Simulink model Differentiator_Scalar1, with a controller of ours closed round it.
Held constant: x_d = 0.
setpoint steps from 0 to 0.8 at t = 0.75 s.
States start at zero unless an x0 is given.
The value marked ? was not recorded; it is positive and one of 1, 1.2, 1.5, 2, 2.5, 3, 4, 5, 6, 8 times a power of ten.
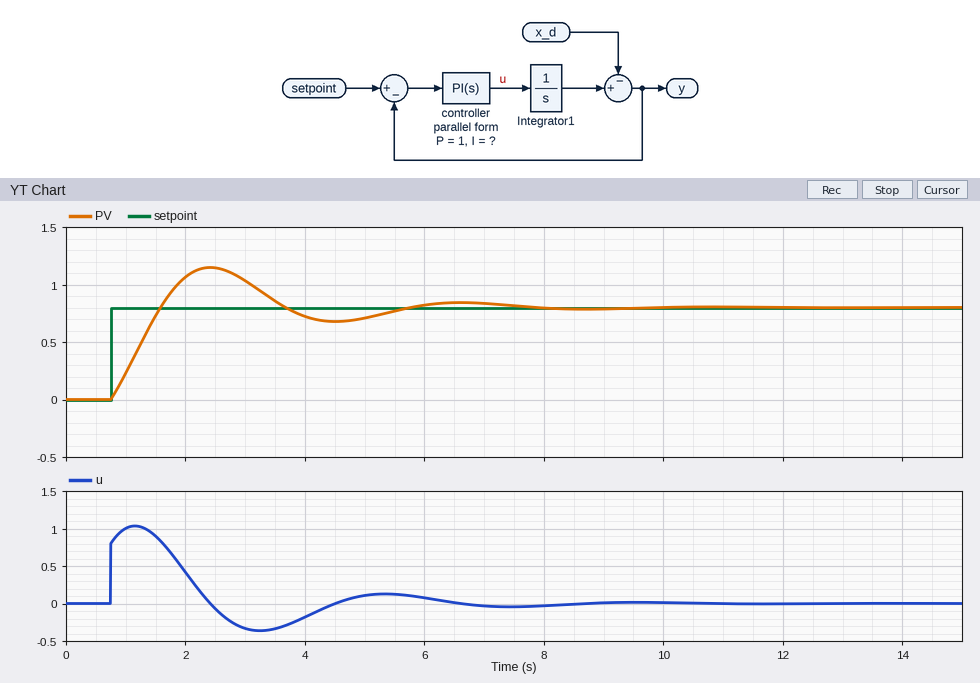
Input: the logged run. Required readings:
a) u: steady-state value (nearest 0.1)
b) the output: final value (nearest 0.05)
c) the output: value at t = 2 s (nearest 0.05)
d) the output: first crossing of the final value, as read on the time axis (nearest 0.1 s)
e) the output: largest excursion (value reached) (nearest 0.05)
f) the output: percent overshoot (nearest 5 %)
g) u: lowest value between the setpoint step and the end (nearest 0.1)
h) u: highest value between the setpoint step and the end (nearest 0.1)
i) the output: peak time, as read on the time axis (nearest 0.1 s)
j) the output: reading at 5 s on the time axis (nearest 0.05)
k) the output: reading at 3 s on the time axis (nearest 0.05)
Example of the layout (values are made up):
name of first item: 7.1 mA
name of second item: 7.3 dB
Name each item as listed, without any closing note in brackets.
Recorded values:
u: steady-state value: 0.0
the output: final value: 0.80
the output: value at t = 2 s: 1.05
the output: first crossing of the final value, as read on the time axis: 1.6 s
the output: largest excursion (value reached): 1.15
the output: percent overshoot: 45 %
u: lowest value between the setpoint step and the end: -0.4
u: highest value between the setpoint step and the end: 1.0
the output: peak time, as read on the time axis: 2.4 s
the output: reading at 5 s on the time axis: 0.70
the output: reading at 3 s on the time axis: 1.05
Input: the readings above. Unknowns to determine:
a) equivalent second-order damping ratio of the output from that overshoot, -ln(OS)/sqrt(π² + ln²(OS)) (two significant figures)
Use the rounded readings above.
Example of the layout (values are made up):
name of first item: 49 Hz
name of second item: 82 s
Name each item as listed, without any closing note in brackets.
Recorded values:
equivalent second-order damping ratio of the output from that overshoot, -ln(OS)/sqrt(π² + ln²(OS)): 0.25
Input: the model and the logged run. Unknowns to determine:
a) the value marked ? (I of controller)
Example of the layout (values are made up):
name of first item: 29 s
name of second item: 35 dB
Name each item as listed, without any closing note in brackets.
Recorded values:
the value marked ?: 2.5
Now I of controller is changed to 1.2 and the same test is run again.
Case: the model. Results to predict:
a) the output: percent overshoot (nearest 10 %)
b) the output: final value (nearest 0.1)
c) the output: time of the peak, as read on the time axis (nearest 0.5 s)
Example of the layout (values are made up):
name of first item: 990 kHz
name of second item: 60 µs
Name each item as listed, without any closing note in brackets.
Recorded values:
the output: percent overshoot: 30 %
the output: final value: 0.8
the output: time of the peak, as read on the time axis: 3.0 s
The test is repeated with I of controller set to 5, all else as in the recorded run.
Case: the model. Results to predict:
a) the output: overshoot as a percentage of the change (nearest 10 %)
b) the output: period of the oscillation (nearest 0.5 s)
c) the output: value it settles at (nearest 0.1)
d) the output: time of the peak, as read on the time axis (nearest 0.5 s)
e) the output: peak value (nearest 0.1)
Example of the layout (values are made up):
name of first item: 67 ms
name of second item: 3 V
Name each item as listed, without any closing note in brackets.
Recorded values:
the output: overshoot as a percentage of the change: 50 %
the output: period of the oscillation: 3.0 s
the output: value it settles at: 0.8
the output: time of the peak, as read on the time axis: 2.0 s
the output: peak value: 1.2
